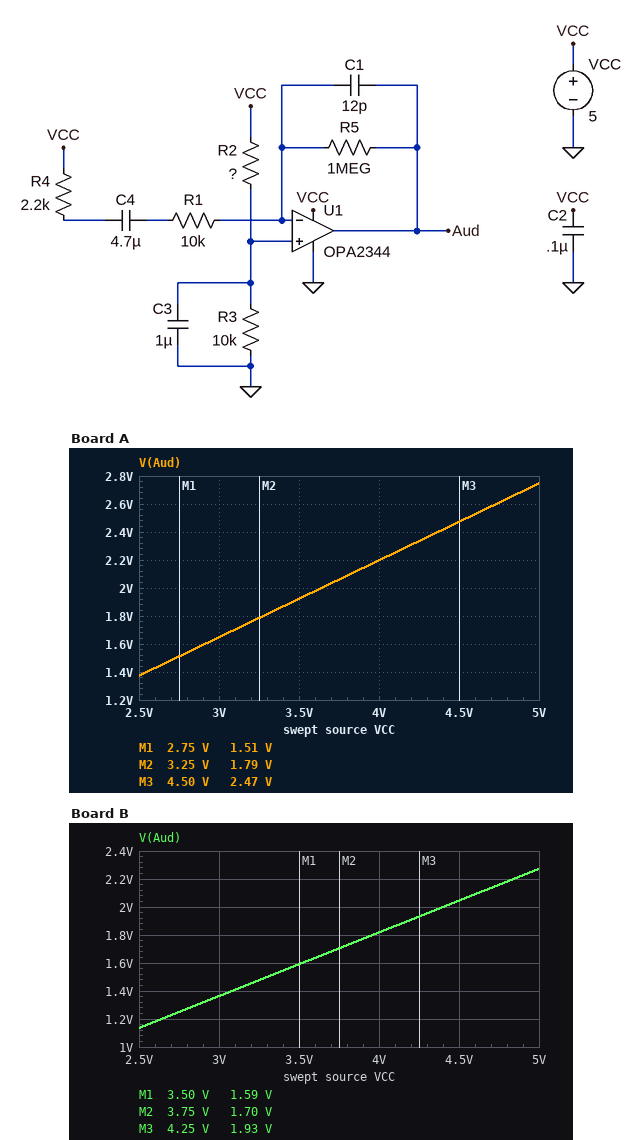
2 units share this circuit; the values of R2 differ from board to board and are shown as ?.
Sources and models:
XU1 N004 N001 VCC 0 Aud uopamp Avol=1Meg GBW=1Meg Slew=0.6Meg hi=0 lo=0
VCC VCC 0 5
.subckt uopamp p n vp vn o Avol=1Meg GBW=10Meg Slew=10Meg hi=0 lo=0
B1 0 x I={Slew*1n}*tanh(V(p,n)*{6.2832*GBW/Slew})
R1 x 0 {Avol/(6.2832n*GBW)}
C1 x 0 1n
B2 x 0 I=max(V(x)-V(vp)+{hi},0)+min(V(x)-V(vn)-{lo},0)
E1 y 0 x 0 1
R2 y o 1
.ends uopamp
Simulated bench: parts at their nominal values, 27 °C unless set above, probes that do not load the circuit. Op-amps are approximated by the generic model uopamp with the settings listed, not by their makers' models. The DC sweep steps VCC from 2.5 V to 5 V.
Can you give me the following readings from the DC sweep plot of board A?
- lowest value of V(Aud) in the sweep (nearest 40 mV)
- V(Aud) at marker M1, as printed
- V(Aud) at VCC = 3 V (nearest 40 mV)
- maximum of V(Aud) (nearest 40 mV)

1.36 V
1.51 V
1.64 V
2.76 V
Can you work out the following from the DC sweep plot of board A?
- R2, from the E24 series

8.2 kΩ
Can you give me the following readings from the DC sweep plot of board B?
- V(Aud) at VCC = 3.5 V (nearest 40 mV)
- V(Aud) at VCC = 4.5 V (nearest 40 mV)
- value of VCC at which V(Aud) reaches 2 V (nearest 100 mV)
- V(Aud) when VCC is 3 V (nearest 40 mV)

1.60 V
2.04 V
4.4 V
1.36 V
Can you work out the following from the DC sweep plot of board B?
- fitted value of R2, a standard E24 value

12 kΩ
